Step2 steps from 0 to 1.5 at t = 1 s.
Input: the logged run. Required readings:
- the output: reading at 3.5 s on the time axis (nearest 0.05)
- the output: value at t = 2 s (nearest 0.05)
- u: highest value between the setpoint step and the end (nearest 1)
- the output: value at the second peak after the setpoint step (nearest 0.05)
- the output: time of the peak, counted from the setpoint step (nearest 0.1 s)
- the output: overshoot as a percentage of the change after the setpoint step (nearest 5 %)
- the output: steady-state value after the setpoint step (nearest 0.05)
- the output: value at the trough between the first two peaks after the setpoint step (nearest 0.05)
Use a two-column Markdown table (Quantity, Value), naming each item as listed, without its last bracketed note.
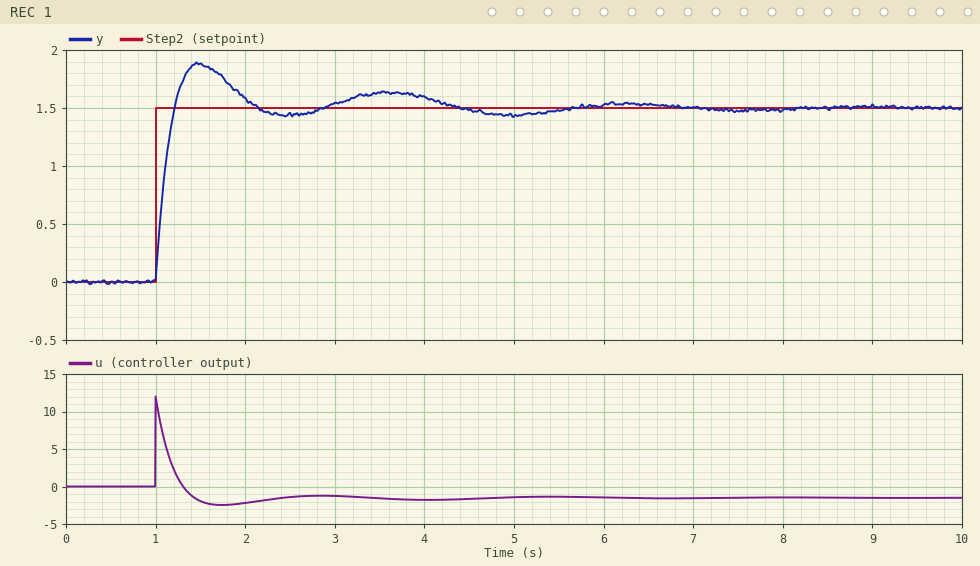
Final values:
| Quantity | Value |
|---|---|
| the output: reading at 3.5 s on the time axis | 1.65 |
| the output: value at t = 2 s | 1.60 |
| u: highest value between the setpoint step and the end | 12 |
| the output: value at the second peak after the setpoint step | 1.65 |
| the output: time of the peak, counted from the setpoint step | 0.5 s |
| the output: overshoot as a percentage of the change after the setpoint step | 25 % |
| the output: steady-state value after the setpoint step | 1.50 |
| the output: value at the trough between the first two peaks after the setpoint step | 1.45 |
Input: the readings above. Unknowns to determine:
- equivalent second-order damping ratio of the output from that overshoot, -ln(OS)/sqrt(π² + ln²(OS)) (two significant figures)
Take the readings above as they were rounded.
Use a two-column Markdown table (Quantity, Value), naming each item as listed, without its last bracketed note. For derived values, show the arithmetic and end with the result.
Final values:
| Quantity | Value |
|---|---|
| equivalent second-order damping ratio of the output from that overshoot, -ln(OS)/sqrt(π² + ln²(OS)) | ln(0.25) = -1.386; 1.386 / sqrt(9.870 + 1.922) = 0.40 |
